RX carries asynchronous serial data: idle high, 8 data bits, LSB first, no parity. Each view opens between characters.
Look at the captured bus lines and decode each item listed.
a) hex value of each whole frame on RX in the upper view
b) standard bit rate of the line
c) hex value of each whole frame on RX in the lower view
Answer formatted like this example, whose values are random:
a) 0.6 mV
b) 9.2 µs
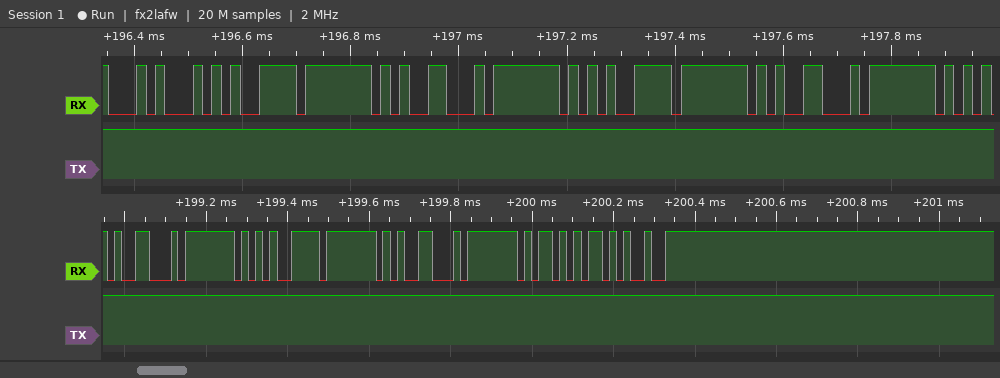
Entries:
a) 14, E5, 7F, 19, 7F, E5, 7F, 19, 7F
b) 57600 baud
c) 19, 7F, E5, 7F, 19, 7F, AB, 25
